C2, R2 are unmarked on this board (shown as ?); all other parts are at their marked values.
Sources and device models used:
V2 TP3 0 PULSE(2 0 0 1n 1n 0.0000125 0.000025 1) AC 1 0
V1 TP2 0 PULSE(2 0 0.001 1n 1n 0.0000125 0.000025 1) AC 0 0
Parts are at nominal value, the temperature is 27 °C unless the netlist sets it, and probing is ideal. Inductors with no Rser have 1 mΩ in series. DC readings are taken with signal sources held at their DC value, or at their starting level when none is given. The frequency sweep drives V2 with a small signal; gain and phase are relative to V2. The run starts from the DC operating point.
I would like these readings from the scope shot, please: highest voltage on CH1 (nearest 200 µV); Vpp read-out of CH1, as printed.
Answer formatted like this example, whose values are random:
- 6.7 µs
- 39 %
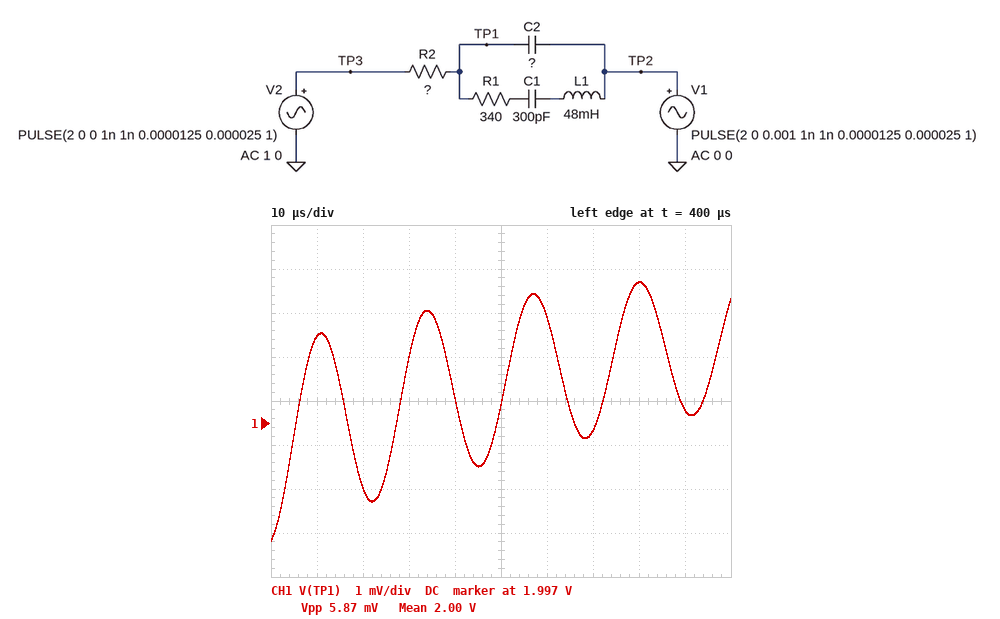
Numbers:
- 2.0002 V
- 5.87 mV
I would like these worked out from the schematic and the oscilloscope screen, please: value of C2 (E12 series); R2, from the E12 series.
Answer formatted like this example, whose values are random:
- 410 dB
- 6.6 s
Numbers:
- 4.7 nF
- 18 kΩ
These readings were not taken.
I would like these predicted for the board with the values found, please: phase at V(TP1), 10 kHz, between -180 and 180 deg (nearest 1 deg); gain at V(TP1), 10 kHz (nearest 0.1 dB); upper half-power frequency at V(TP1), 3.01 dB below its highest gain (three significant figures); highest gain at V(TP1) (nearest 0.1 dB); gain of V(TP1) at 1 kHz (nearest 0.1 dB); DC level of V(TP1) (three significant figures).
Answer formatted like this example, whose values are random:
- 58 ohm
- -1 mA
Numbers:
- -80 deg
- -15.2 dB
- 1.77 kHz
- 0 dB
- -1.2 dB
- 2.00 V
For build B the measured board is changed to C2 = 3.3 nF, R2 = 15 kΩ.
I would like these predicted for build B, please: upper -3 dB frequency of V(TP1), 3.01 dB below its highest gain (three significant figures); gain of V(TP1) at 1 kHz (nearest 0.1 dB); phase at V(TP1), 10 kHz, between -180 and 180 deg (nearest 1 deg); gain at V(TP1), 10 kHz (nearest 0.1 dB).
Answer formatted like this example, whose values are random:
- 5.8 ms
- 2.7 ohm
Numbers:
- 2.95 kHz
- -0.5 dB
- -74 deg
- -11.0 dB
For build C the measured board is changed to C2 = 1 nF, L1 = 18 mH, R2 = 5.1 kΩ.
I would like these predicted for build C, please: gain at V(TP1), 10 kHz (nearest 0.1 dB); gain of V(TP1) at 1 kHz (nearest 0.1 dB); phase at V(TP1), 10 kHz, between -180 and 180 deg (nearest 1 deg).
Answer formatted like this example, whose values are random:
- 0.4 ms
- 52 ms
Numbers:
- -0.7 dB
- 0 dB
- -23 deg
